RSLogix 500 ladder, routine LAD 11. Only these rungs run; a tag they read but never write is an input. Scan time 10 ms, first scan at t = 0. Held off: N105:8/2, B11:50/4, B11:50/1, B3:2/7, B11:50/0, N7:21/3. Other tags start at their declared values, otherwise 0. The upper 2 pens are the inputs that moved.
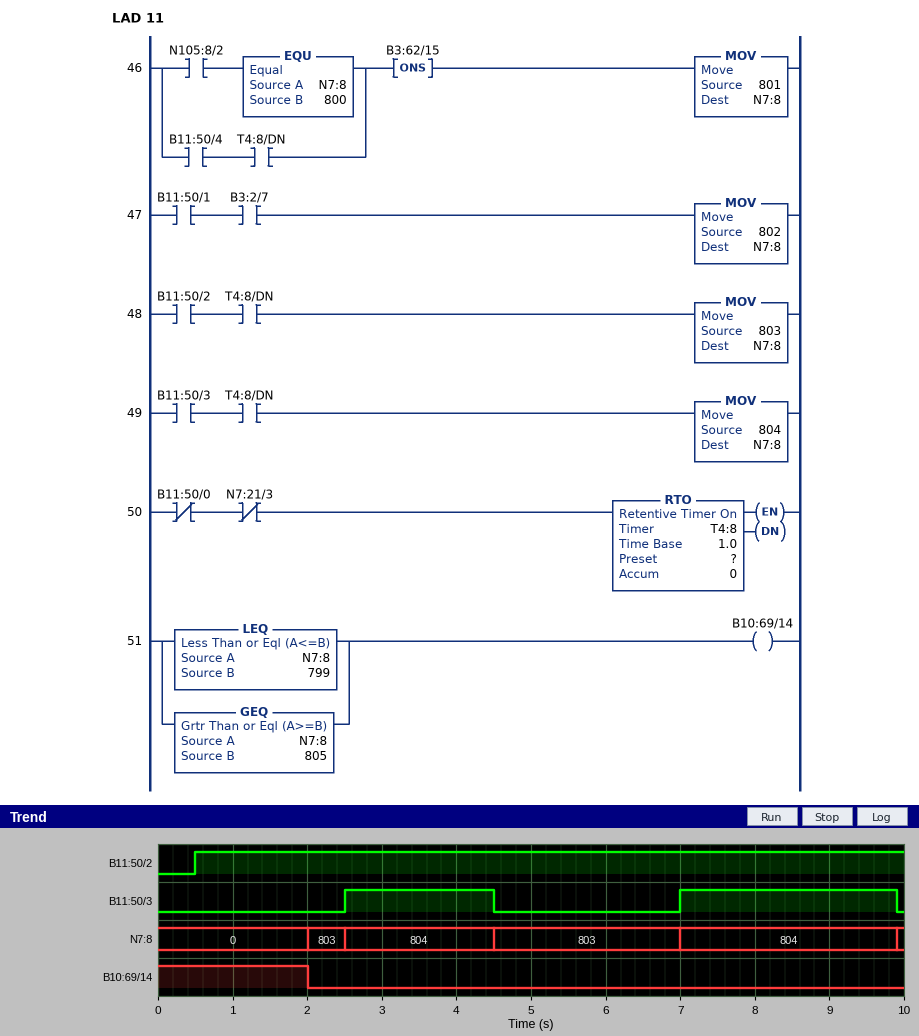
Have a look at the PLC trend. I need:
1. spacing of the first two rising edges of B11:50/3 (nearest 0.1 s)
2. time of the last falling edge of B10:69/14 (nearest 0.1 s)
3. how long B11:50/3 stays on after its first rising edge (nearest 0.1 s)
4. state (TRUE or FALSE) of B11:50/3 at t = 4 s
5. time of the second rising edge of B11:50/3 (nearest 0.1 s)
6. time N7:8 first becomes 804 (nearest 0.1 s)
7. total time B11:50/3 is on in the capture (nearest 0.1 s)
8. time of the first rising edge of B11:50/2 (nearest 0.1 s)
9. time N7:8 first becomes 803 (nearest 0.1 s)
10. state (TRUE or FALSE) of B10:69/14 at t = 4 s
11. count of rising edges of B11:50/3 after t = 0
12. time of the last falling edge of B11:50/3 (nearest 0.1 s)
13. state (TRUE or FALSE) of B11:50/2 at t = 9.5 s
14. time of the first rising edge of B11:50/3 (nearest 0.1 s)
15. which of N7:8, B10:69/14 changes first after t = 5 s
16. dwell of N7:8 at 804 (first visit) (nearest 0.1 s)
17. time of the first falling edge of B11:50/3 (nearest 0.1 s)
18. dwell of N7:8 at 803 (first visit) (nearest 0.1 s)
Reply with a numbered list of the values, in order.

1. 4.5 s
2. 2.0 s
3. 2.0 s
4. TRUE
5. 7.0 s
6. 2.5 s
7. 4.9 s
8. 0.5 s
9. 2.0 s
10. FALSE
11. 2
12. 9.9 s
13. TRUE
14. 2.5 s
15. N7:8
16. 2.0 s
17. 4.5 s
18. 0.5 s
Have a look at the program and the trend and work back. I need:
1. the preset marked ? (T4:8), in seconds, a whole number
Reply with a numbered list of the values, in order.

1. 2 s
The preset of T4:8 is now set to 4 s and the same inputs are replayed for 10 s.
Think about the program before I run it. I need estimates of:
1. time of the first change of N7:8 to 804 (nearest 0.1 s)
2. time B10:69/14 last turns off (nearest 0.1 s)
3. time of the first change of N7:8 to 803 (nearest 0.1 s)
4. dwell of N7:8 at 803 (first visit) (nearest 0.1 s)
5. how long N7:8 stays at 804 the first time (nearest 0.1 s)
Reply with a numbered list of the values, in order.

1. 4.0 s
2. 4.0 s
3. 4.5 s
4. 2.5 s
5. 0.5 s
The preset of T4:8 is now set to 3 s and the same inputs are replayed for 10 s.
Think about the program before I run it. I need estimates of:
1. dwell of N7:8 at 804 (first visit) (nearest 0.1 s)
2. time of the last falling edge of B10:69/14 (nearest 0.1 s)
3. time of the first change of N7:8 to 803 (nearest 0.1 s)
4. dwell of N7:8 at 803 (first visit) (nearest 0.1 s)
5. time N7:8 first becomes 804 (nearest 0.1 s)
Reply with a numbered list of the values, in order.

1. 1.5 s
2. 3.0 s
3. 4.5 s
4. 2.5 s
5. 3.0 s
